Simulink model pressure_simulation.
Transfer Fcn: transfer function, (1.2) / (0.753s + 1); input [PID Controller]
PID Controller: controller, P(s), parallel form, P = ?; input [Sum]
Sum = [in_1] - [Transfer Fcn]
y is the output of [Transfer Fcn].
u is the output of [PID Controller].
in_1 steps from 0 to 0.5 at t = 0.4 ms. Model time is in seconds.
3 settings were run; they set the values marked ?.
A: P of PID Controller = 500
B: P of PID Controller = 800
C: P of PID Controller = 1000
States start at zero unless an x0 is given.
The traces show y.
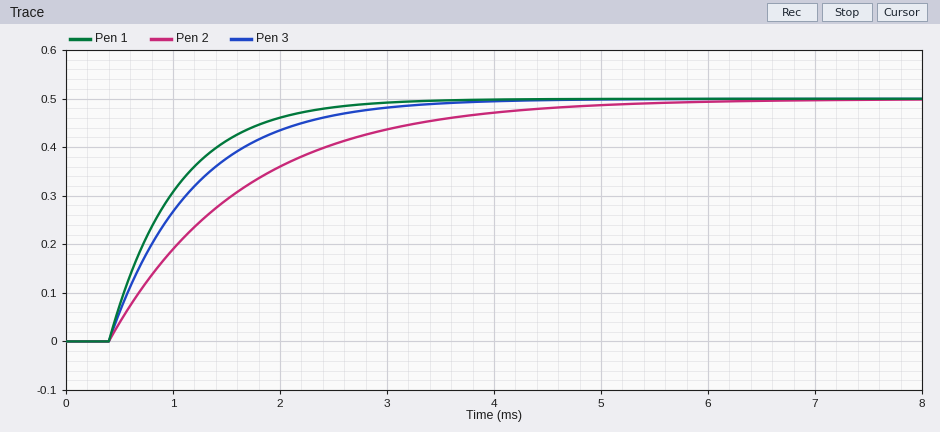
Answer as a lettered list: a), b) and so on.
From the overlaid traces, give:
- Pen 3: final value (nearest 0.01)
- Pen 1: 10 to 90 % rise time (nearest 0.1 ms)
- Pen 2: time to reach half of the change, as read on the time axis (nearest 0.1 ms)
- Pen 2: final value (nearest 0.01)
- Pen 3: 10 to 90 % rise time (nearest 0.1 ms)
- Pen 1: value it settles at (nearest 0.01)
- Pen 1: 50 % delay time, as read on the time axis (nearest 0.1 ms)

a) 0.50
b) 1.4 ms
c) 1.3 ms
d) 0.50
e) 1.7 ms
f) 0.50
g) 0.8 ms
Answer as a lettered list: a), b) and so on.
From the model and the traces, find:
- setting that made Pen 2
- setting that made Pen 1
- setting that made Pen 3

a) A
b) C
c) B
